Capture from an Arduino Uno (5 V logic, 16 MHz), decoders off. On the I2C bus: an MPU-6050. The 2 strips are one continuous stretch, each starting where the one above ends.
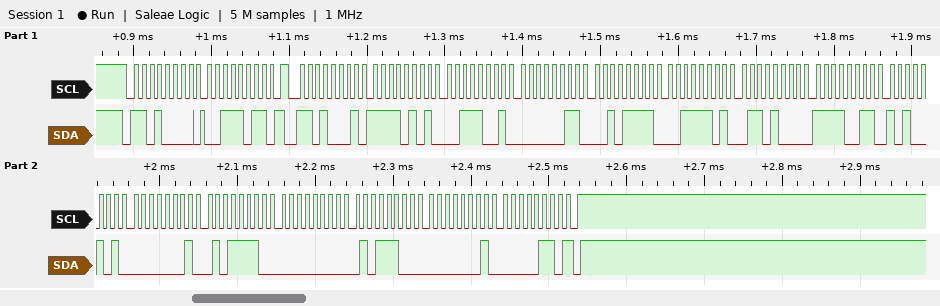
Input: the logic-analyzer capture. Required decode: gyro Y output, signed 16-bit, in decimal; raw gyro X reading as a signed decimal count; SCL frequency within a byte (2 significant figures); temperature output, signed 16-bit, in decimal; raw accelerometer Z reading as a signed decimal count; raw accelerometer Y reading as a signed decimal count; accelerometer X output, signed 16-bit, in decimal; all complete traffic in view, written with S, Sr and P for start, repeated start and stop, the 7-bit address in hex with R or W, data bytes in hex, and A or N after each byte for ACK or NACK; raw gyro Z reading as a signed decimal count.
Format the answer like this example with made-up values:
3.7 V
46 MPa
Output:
92
350
100 kHz
-3163
15720
815
-2759
S 68W A 3B A Sr 68R A F5 A 39 A 03 A 2F A 3D A 68 A F3 A A5 A 01 A 5E A 00 A 5C A 01 A 06 N P
262
